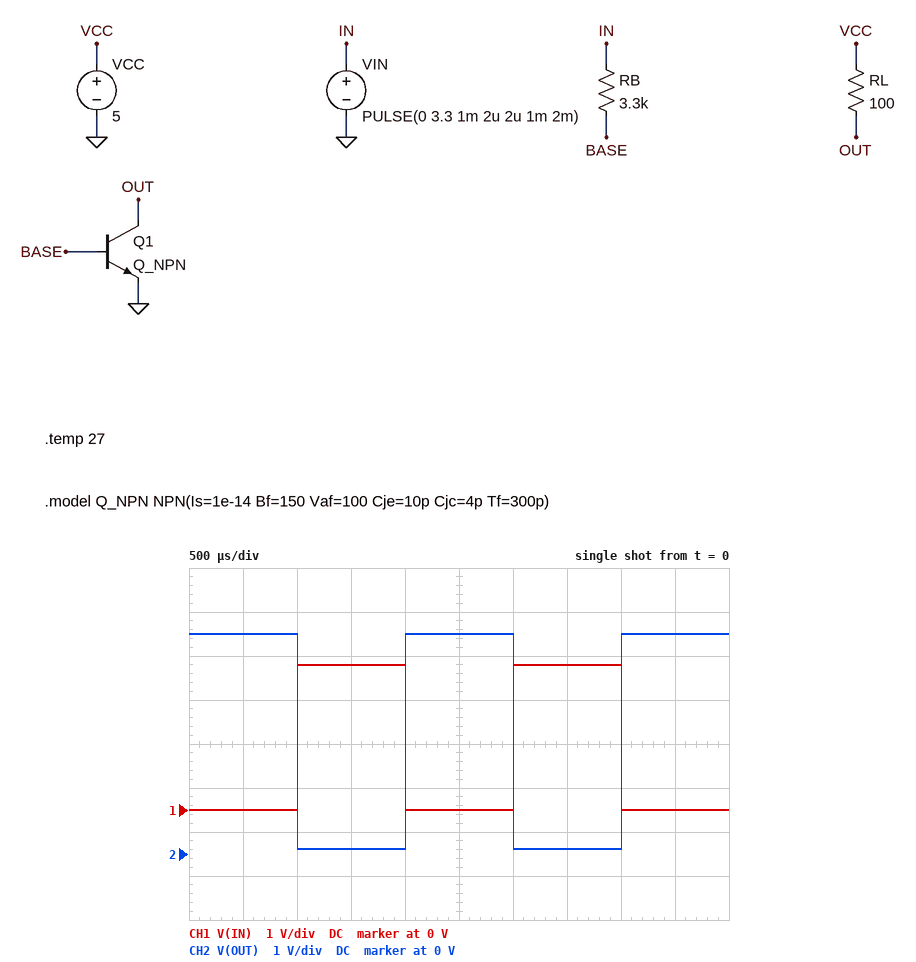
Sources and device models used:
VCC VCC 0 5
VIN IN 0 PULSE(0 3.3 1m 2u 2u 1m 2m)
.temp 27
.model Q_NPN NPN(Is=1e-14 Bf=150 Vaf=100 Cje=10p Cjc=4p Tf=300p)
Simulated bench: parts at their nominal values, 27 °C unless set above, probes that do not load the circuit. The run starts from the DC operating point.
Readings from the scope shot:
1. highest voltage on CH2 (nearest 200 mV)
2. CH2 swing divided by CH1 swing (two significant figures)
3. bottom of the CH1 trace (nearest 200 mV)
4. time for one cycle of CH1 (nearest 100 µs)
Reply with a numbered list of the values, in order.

1. 5.0 V
2. 1.5
3. 0 V
4. 2.0 ms
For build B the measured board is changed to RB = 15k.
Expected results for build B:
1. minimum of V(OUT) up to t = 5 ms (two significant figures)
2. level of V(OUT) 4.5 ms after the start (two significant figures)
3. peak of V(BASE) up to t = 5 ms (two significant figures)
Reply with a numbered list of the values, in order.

1. 2.4 V
2. 5.0 V
3. 740 mV
